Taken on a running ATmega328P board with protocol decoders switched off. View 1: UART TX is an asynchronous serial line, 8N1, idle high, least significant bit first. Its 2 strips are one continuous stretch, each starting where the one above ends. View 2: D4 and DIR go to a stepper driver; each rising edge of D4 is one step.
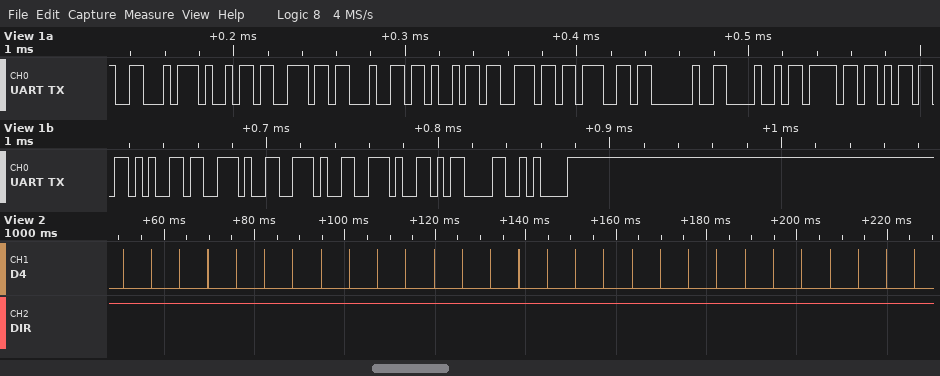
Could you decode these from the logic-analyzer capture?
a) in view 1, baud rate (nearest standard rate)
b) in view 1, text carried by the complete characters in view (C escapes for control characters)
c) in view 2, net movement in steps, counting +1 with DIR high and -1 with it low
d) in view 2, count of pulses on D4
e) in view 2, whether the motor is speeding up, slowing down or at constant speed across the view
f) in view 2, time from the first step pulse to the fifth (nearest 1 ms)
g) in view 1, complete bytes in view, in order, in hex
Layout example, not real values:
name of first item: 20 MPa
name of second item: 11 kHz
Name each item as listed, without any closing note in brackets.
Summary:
in view 1, baud rate: 250000 baud
in view 1, text carried by the complete characters in view: "Finding Home...\r\n"
in view 2, net movement in steps, counting +1 with DIR high and -1 with it low: +29
in view 2, count of pulses on D4: 29
in view 2, whether the motor is speeding up, slowing down or at constant speed across the view: constant speed
in view 2, time from the first step pulse to the fifth: 25 ms
in view 1, complete bytes in view, in order, in hex: 46 69 6E 64 69 6E 67 20 48 6F 6D 65 2E 2E 2E 0D 0A
